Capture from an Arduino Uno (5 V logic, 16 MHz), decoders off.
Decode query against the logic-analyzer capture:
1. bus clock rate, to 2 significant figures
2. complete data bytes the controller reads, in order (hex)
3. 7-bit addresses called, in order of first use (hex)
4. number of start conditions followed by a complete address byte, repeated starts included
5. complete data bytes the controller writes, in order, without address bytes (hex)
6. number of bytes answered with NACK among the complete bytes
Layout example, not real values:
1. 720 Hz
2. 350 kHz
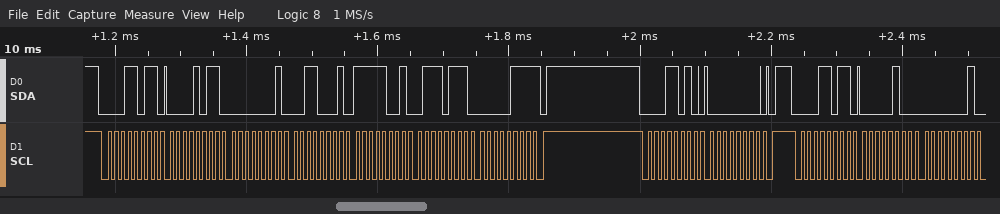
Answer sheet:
1. 100 kHz
2. 0B 01 31 F9 77 07 04 01
3. 0x0D
4. 3
5. 00
6. 1
